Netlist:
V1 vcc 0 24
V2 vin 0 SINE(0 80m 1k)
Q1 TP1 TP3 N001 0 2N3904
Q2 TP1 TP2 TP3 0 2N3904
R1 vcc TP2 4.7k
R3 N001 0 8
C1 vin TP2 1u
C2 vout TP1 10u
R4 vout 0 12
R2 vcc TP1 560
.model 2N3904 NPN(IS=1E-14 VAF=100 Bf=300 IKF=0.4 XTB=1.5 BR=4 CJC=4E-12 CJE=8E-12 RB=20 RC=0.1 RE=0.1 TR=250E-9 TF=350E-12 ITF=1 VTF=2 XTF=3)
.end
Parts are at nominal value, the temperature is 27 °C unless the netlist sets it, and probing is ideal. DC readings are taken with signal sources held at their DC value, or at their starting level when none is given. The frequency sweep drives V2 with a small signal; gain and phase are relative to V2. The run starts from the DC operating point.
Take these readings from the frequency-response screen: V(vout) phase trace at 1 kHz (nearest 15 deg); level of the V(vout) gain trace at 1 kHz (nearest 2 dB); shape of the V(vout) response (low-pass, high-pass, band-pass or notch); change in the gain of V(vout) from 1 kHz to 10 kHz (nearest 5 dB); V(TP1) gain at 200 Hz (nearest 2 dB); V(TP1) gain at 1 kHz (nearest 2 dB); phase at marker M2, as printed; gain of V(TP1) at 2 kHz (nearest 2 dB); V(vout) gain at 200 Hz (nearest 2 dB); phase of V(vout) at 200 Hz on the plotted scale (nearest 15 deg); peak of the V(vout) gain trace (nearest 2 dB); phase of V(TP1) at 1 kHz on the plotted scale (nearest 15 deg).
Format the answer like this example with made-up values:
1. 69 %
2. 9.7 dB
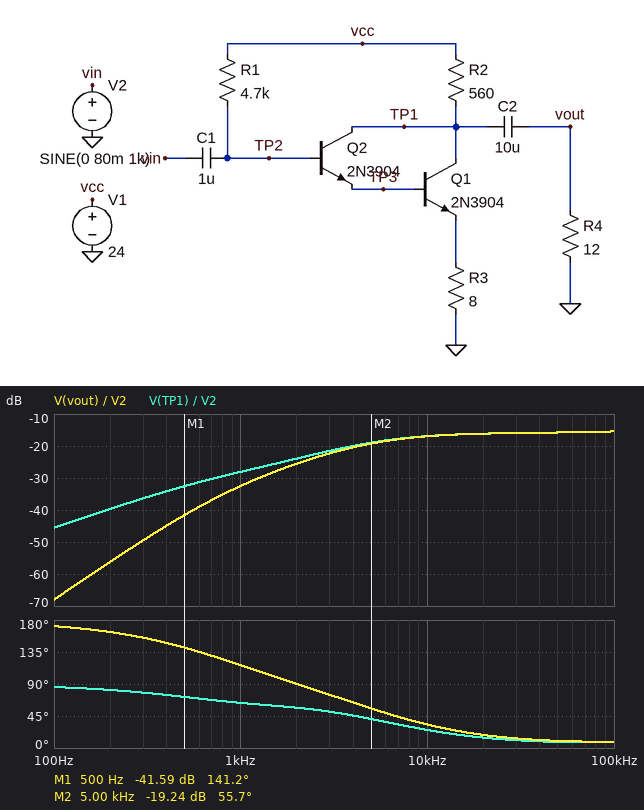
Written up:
1. 120 deg
2. -32 dB
3. high-pass
4. 15 dB
5. -40 dB
6. -28 dB
7. 55.7 deg
8. -24 dB
9. -56 dB
10. 165 deg
11. -16 dB
12. 60 deg
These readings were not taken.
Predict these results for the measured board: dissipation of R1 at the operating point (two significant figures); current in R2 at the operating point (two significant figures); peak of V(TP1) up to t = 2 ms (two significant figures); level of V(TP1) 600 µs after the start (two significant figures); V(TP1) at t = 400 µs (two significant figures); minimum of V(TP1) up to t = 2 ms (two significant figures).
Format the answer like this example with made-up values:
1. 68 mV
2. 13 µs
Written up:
1. 100 mW
2. 41 mA
3. 1.1 V
4. 1.1 V
5. 1.1 V
6. 1.1 V
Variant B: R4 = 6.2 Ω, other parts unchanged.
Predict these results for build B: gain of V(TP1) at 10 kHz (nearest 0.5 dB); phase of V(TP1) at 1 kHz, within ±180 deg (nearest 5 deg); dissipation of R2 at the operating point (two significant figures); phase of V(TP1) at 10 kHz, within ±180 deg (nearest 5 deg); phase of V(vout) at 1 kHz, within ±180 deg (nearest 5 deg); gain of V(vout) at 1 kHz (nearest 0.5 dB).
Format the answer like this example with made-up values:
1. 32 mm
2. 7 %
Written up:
1. -19.5 dB
2. 55 deg
3. 930 mW
4. 20 deg
5. 125 deg
6. -36.5 dB
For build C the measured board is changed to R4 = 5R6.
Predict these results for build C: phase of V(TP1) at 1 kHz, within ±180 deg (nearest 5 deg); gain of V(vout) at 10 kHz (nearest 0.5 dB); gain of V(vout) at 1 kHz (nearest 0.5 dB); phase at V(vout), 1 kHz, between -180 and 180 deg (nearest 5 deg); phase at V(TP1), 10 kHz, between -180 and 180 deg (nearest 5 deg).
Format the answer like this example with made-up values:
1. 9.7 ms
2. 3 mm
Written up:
1. 55 deg
2. -20.0 dB
3. -37.5 dB
4. 125 deg
5. 20 deg
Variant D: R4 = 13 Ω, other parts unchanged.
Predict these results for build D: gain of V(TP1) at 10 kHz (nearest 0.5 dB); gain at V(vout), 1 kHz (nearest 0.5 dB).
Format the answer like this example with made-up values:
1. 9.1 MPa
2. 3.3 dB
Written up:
1. -16.5 dB
2. -32.0 dB
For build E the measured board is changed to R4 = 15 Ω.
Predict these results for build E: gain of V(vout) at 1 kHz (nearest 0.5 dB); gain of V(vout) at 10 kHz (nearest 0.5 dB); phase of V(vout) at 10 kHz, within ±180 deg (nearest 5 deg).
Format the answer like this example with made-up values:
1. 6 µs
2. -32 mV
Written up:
1. -31.5 dB
2. -16.5 dB
3. 30 deg
